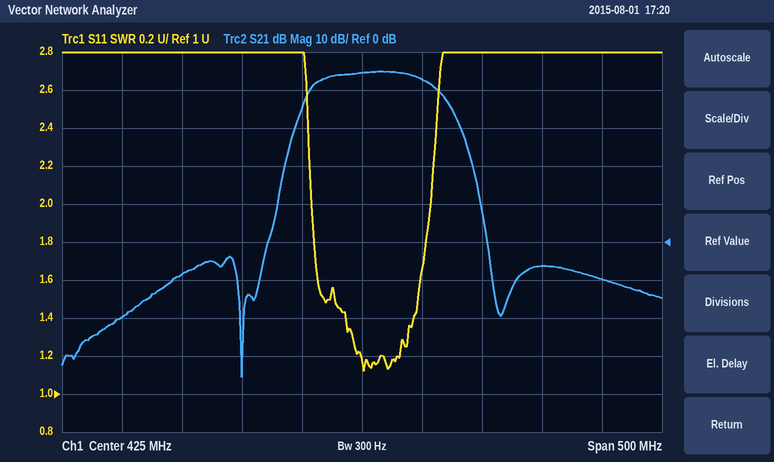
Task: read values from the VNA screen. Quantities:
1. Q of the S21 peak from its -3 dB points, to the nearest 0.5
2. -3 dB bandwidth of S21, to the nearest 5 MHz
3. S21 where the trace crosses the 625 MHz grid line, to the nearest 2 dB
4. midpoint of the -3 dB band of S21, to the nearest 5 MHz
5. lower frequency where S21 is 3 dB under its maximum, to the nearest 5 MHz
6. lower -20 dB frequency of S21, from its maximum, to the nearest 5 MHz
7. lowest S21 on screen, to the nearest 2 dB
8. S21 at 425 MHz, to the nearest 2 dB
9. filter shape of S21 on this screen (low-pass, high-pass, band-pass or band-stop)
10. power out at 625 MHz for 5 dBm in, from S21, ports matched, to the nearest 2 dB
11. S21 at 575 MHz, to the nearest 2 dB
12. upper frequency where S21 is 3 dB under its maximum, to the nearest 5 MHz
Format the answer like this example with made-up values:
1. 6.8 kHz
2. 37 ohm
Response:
1. 4.5
2. 95 MHz
3. -10 dB
4. 435 MHz
5. 385 MHz
6. 365 MHz
7. -36 dB
8. 44 dB
9. band-pass
10. -4 dBm
11. -6 dB
12. 480 MHz
